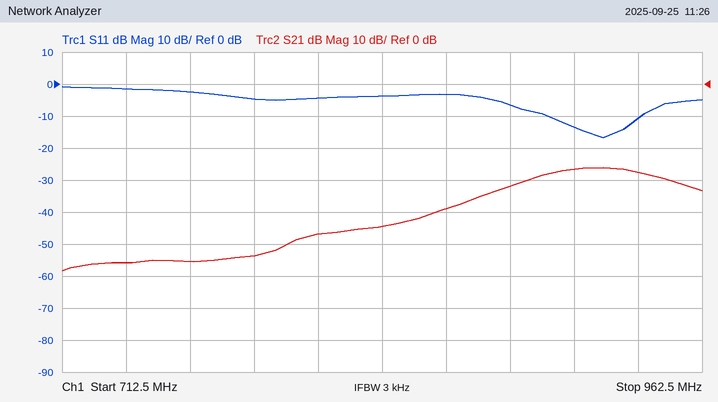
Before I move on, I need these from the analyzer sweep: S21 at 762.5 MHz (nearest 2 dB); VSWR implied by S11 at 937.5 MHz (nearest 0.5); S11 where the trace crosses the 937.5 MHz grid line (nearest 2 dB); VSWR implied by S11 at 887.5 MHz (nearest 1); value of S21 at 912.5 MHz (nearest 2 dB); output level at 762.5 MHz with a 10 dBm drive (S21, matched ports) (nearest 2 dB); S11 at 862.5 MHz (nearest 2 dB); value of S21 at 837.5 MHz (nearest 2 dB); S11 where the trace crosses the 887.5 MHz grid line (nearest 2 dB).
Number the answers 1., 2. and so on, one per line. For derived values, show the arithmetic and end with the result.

1. -56 dB
2. |Γ| = 10^(-10/20) = 0.3162; VSWR = (1 + 0.3162)/(1 − 0.3162) ≈ 1.92, so 2.0 to the nearest 0.5
3. -10 dB
4. |Γ| = 10^(-6/20) = 0.5012; VSWR = (1 + 0.5012)/(1 − 0.5012) ≈ 3
5. -26 dB
6. 10 dBm + (-56 dB) = -46 dBm
7. -4 dB
8. -44 dB
9. -6 dB
